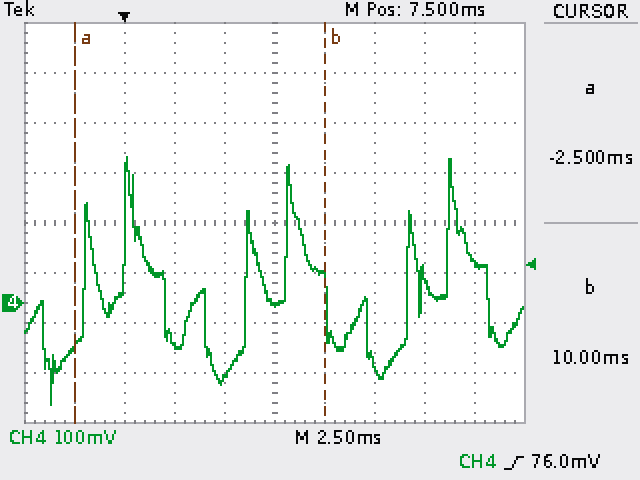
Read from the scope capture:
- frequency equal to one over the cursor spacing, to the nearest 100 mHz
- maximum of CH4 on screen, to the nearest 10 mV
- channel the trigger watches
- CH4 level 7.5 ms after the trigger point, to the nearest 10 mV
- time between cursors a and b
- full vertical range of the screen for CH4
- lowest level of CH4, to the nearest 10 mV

80.0 Hz
290 mV
CH4
0 mV
12.50 ms
800 mV
-200 mV
